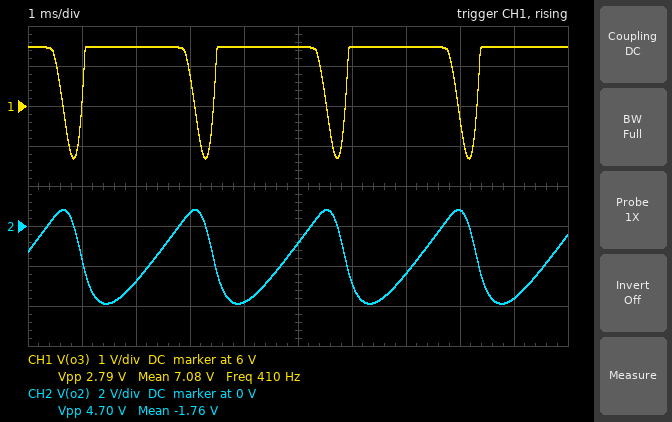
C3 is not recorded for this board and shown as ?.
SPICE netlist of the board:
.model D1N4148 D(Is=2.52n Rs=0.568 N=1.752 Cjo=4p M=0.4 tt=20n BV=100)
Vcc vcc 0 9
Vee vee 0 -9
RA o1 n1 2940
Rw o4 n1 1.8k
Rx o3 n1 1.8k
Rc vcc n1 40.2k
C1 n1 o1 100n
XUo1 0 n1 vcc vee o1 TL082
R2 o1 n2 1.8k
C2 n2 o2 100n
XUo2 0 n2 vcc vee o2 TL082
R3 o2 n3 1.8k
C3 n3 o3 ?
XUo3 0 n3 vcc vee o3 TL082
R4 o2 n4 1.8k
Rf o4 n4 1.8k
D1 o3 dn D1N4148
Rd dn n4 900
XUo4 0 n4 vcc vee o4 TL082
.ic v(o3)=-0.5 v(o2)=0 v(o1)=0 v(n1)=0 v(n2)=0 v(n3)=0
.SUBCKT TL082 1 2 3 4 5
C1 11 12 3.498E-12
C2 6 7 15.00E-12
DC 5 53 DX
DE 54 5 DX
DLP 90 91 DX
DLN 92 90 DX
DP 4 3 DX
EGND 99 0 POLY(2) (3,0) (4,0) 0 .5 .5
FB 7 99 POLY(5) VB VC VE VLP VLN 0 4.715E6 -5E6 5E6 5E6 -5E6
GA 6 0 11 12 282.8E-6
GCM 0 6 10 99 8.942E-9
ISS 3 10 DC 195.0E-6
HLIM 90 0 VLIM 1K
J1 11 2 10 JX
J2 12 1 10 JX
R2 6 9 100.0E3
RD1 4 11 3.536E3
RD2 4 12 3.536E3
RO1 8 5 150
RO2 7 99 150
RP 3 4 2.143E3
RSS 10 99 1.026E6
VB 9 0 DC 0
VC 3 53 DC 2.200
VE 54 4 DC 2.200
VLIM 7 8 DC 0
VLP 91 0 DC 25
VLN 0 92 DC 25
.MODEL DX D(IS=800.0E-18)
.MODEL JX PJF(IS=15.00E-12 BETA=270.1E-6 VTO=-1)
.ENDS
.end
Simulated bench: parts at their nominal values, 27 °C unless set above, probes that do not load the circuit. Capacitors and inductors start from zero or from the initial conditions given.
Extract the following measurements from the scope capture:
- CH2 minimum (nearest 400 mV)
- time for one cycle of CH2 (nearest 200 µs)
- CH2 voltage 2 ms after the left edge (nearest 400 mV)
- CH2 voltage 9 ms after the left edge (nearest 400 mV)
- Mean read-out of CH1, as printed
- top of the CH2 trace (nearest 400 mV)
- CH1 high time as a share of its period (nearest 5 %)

-4.0 V
2.4 ms
-2.8 V
-3.6 V
7.08 V
800 mV
85 %
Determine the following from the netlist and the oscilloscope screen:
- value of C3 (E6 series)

47 nF
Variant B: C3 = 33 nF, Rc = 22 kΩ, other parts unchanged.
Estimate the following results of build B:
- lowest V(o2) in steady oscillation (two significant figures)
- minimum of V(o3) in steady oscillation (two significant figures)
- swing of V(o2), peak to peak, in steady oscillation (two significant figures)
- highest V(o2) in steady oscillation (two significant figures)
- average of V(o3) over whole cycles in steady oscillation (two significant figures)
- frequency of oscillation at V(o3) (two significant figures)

-2.2 V
1.9 V
3.3 V
1.2 V
5.8 V
620 Hz
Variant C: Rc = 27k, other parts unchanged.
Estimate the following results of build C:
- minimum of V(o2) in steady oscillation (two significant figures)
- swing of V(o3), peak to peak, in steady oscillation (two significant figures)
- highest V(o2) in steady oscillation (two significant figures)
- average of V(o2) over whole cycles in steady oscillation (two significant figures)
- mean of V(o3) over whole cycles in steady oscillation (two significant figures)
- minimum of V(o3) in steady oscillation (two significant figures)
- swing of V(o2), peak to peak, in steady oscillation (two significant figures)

-3.7 V
4.2 V
1.2 V
-1.5 V
6.6 V
3.3 V
4.9 V
